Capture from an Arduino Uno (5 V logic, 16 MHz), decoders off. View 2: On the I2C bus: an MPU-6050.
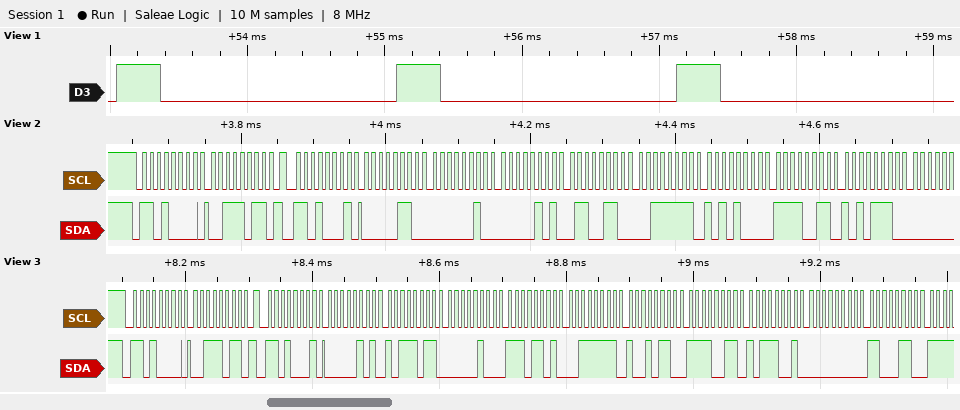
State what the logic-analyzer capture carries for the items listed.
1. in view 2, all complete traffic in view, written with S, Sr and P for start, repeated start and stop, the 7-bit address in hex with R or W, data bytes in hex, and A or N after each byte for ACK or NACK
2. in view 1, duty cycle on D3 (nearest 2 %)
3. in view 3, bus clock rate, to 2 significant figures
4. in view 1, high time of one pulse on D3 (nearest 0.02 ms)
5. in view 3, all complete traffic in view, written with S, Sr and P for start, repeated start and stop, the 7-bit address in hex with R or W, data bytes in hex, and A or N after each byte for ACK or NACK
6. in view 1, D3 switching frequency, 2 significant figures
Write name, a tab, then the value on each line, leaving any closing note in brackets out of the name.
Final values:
in view 2, all complete traffic in view, written with S, Sr and P for start, repeated start and stop, the 7-bit address in hex with R or W, data bytes in hex, and A or N after each byte for ACK or NACK	S 68W A 3B A Sr 68R A 06 A 02 A 05 A 66 A 3F A A8 A F3 A AE A
in view 1, duty cycle on D3	16 %
in view 3, bus clock rate, to 2 significant figures	100 kHz
in view 1, high time of one pulse on D3	0.32 ms
in view 3, all complete traffic in view, written with S, Sr and P for start, repeated start and stop, the 7-bit address in hex with R or W, data bytes in hex, and A or N after each byte for ACK or NACK	S 68W A 3B A Sr 68R A 05 A BB A 04 A ED A 3F A 96 A F3 A B9 A 00 A C6 A
in view 1, D3 switching frequency, 2 significant figures	490 Hz
